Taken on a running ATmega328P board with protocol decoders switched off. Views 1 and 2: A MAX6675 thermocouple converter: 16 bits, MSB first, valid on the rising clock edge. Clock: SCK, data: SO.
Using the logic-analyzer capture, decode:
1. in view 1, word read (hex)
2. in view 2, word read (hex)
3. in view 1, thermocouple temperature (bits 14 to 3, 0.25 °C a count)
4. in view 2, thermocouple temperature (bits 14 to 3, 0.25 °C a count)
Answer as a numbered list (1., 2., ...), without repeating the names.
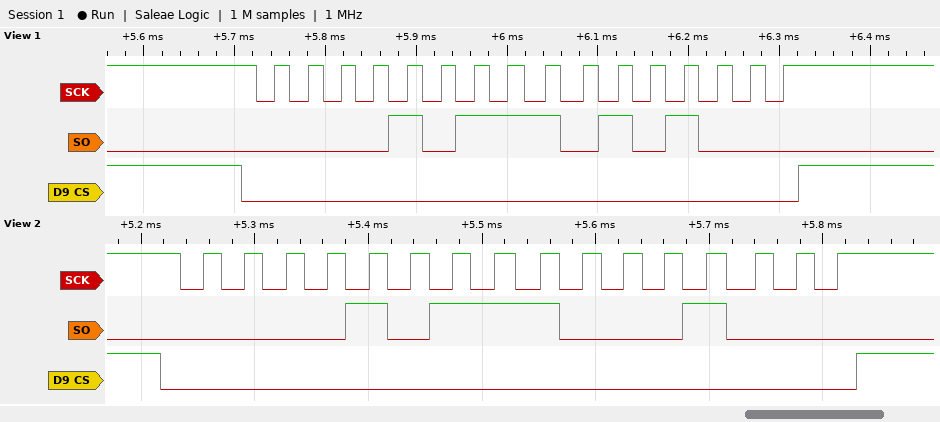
1. 0x0BA8
2. 0x0B88
3. 93.25 °C
4. 92.25 °C
